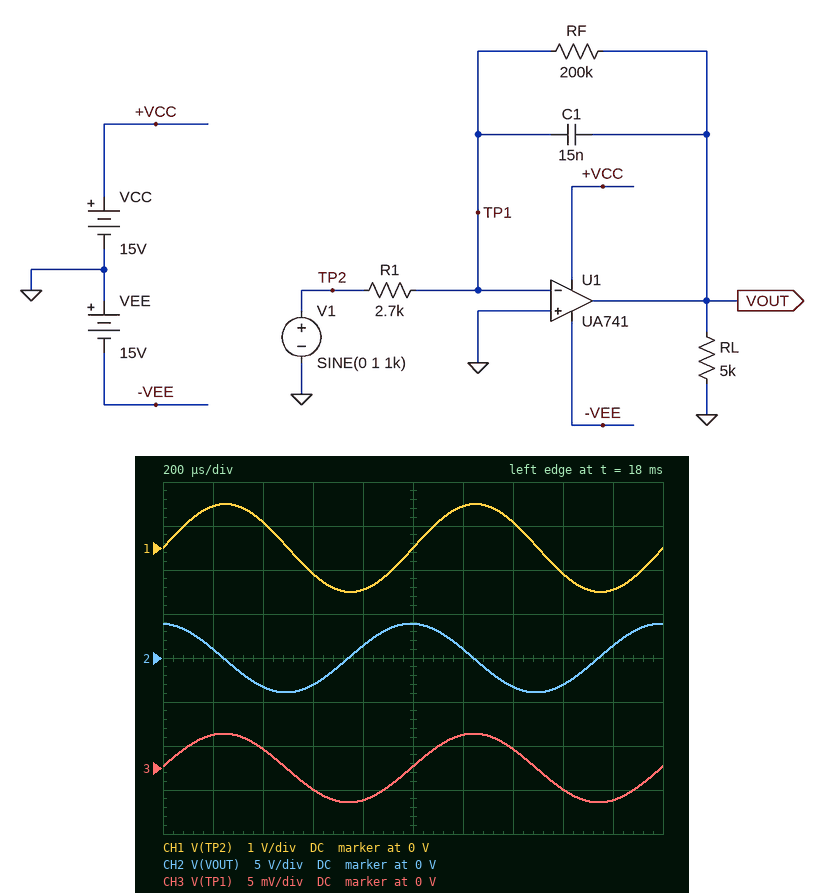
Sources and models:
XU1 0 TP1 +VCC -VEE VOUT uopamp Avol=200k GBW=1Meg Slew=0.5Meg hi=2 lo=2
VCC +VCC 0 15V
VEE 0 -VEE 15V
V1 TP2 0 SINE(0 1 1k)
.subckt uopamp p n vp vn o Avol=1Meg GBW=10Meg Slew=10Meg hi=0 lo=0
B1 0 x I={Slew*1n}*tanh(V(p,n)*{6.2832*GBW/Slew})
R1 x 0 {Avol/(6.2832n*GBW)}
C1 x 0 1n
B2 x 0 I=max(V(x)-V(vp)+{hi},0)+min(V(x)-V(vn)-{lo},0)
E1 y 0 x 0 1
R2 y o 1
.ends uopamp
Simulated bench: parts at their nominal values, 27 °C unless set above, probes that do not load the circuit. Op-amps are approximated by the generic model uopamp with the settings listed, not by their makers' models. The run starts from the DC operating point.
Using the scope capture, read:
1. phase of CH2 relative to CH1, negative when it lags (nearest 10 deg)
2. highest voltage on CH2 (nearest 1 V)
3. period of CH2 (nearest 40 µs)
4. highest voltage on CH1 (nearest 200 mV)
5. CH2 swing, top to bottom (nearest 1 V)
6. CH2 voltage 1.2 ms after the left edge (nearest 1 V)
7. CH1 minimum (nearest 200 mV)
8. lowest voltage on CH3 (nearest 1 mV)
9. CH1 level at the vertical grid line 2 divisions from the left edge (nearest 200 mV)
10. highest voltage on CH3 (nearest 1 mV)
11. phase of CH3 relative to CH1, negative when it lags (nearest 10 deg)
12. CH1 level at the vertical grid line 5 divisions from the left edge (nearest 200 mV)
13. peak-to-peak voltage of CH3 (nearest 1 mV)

90 deg
4 V
1.00 ms
1.0 V
8 V
1 V
-1.0 V
-4 mV
600 mV
4 mV
0 deg
0 V
8 mV
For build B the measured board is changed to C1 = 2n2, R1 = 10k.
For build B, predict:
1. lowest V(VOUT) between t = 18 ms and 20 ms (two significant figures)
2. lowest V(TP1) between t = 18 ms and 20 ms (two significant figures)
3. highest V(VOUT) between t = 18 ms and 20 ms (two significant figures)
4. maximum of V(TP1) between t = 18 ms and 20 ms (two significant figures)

-6.8 V
-6.8 mV
6.8 V
6.8 mV
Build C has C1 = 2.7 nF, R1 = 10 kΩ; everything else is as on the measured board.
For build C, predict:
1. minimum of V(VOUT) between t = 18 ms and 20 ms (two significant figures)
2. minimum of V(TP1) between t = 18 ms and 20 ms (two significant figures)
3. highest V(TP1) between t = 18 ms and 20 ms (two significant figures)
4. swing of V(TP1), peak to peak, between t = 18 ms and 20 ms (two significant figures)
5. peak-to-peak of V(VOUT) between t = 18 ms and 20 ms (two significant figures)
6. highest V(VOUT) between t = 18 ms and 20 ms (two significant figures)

-5.6 V
-5.6 mV
5.6 mV
11 mV
11 V
5.6 V
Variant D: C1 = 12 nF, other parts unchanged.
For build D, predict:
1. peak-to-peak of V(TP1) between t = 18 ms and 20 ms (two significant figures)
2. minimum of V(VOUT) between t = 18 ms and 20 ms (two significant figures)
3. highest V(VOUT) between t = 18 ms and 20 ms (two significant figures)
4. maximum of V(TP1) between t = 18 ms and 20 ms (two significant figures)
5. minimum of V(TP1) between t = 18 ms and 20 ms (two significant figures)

9.8 mV
-4.9 V
4.9 V
4.9 mV
-4.9 mV
